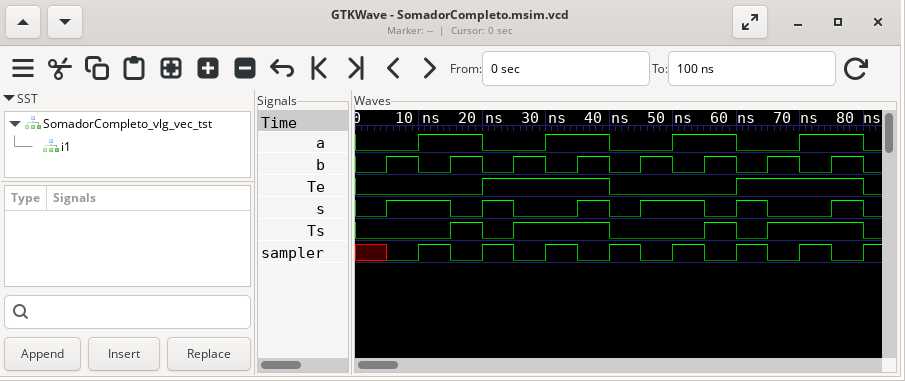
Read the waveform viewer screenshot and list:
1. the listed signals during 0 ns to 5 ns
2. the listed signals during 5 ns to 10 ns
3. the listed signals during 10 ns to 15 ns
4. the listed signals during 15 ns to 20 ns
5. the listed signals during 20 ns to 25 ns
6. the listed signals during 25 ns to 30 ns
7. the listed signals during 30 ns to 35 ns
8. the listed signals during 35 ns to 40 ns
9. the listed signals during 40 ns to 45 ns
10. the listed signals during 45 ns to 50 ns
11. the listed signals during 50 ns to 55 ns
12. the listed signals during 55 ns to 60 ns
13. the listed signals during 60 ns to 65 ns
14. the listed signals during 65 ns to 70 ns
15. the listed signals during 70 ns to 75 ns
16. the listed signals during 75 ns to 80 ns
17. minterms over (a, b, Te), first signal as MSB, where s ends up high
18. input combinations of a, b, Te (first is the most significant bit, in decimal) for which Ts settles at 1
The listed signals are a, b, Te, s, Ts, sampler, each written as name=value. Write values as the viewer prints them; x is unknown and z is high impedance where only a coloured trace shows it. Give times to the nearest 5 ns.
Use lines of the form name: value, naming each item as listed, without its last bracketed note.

the listed signals during 0 ns to 5 ns: a=0, b=0, Te=0, s=0, Ts=0, sampler=x
the listed signals during 5 ns to 10 ns: a=0, b=1, Te=0, s=1, Ts=0, sampler=0
the listed signals during 10 ns to 15 ns: a=1, b=0, Te=0, s=1, Ts=0, sampler=1
the listed signals during 15 ns to 20 ns: a=1, b=1, Te=0, s=0, Ts=1, sampler=0
the listed signals during 20 ns to 25 ns: a=0, b=0, Te=1, s=1, Ts=0, sampler=1
the listed signals during 25 ns to 30 ns: a=0, b=1, Te=1, s=0, Ts=1, sampler=0
the listed signals during 30 ns to 35 ns: a=1, b=0, Te=1, s=0, Ts=1, sampler=1
the listed signals during 35 ns to 40 ns: a=1, b=1, Te=1, s=1, Ts=1, sampler=0
the listed signals during 40 ns to 45 ns: a=0, b=0, Te=0, s=0, Ts=0, sampler=1
the listed signals during 45 ns to 50 ns: a=0, b=1, Te=0, s=1, Ts=0, sampler=0
the listed signals during 50 ns to 55 ns: a=1, b=0, Te=0, s=1, Ts=0, sampler=1
the listed signals during 55 ns to 60 ns: a=1, b=1, Te=0, s=0, Ts=1, sampler=0
the listed signals during 60 ns to 65 ns: a=0, b=0, Te=1, s=1, Ts=0, sampler=1
the listed signals during 65 ns to 70 ns: a=0, b=1, Te=1, s=0, Ts=1, sampler=0
the listed signals during 70 ns to 75 ns: a=1, b=0, Te=1, s=0, Ts=1, sampler=1
the listed signals during 75 ns to 80 ns: a=1, b=1, Te=1, s=1, Ts=1, sampler=0
minterms over (a, b, Te), first signal as MSB, where s ends up high: 1, 2, 4, 7
input combinations of a, b, Te (first is the most significant bit, in decimal) for which Ts settles at 1: 3, 5, 6, 7
